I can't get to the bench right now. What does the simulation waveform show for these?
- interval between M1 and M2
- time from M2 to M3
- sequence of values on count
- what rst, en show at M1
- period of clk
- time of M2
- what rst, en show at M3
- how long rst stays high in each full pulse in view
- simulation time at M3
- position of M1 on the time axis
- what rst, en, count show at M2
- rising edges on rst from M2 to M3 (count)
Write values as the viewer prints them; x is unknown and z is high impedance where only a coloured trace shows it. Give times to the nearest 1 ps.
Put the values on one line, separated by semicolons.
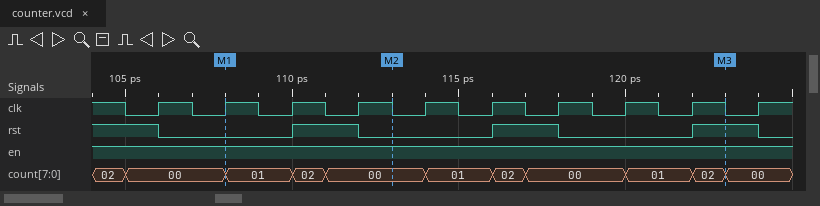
5 ps; 10 ps; 02, 00, 01, 02, 00, 01, 02, 00, 01, 02, 00; rst=0, en=1; 2 ps; 113 ps; rst=1, en=1; 2 ps, 2 ps, 2 ps; 123 ps; 108 ps; rst=0, en=1, count=00; 2
